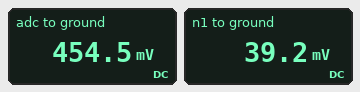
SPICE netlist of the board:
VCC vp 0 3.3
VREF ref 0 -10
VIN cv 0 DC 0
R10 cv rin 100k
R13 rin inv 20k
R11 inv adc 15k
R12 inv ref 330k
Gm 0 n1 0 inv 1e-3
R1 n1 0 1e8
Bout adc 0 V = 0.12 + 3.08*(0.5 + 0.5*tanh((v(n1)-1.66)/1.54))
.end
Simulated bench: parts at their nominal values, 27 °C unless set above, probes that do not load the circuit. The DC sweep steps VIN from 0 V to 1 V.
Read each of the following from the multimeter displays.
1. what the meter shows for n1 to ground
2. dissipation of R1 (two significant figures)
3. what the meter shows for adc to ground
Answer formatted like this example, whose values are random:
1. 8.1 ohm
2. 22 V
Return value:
1. 39.2 mV
2. 15 pW
3. 454.5 mV
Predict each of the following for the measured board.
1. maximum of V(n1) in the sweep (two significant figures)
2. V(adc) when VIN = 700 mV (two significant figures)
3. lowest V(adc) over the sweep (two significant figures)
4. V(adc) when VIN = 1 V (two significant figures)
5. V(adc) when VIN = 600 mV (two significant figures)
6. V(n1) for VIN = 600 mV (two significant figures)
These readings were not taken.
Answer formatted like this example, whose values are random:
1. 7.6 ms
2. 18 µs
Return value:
1. 39 mV
2. 370 mV
3. 330 mV
4. 330 mV
5. 380 mV
6. -180 mV
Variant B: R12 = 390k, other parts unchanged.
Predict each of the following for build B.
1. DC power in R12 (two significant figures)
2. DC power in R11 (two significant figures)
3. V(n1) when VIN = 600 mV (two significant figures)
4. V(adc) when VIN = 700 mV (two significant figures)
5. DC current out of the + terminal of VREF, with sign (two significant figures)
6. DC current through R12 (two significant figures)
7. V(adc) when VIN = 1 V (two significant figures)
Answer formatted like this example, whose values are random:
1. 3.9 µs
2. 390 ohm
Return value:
1. 260 µW
2. 9.9 µW
3. -440 mV
4. 300 mV
5. -26 µA
6. 26 µA
7. 260 mV
